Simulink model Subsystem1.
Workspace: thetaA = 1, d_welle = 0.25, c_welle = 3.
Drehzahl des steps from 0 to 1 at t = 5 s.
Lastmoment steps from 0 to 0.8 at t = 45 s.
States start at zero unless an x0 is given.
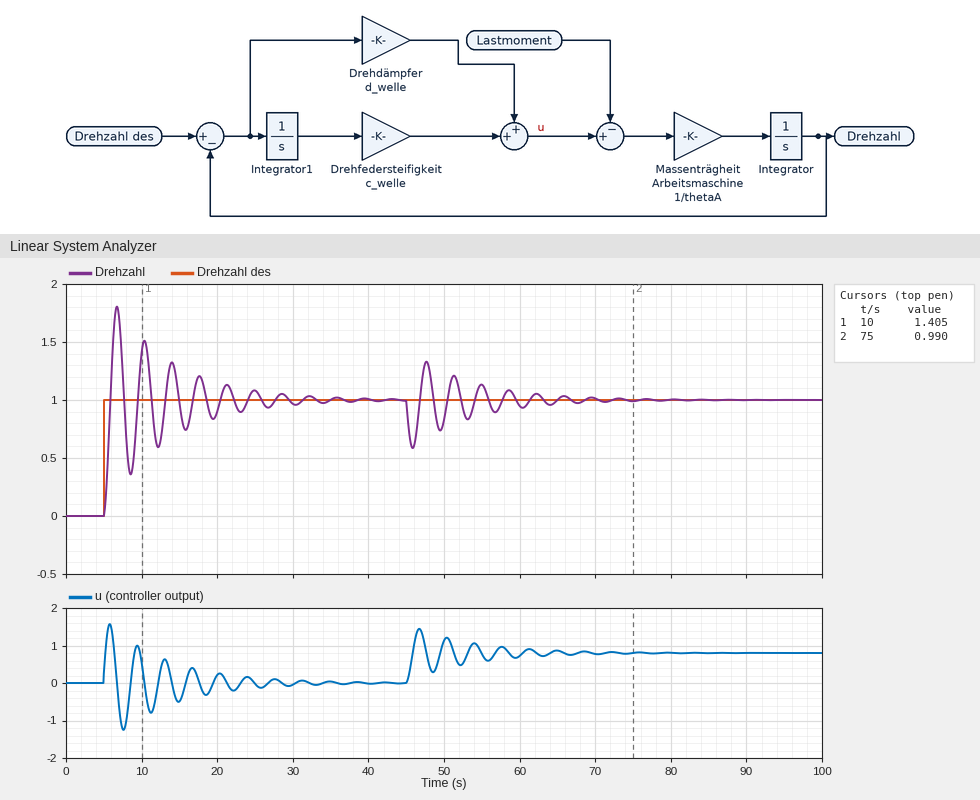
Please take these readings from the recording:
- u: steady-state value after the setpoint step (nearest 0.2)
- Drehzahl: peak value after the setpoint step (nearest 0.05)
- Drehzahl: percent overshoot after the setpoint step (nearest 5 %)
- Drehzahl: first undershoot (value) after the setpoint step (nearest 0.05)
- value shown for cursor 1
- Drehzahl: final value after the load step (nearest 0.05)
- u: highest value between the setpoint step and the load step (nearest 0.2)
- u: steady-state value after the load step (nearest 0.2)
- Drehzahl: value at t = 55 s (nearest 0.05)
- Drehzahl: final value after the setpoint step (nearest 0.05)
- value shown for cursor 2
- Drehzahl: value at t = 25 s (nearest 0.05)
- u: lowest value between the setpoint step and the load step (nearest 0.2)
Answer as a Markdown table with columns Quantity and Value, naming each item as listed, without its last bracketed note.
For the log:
| Quantity | Value |
|---|---|
| u: steady-state value after the setpoint step | 0.0 |
| Drehzahl: peak value after the setpoint step | 1.80 |
| Drehzahl: percent overshoot after the setpoint step | 80 % |
| Drehzahl: first undershoot (value) after the setpoint step | 0.35 |
| value shown for cursor 1 | 1.405 |
| Drehzahl: final value after the load step | 1.00 |
| u: highest value between the setpoint step and the load step | 1.6 |
| u: steady-state value after the load step | 0.8 |
| Drehzahl: value at t = 55 s | 1.15 |
| Drehzahl: final value after the setpoint step | 1.00 |
| value shown for cursor 2 | 0.990 |
| Drehzahl: value at t = 25 s | 1.10 |
| u: lowest value between the setpoint step and the load step | -1.2 |
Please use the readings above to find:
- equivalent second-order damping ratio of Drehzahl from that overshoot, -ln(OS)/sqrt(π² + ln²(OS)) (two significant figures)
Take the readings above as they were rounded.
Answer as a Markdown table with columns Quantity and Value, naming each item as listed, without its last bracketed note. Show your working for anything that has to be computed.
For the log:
| Quantity | Value |
|---|---|
| equivalent second-order damping ratio of Drehzahl from that overshoot, -ln(OS)/sqrt(π² + ln²(OS)) | ln(0.8) = -0.223; 0.223 / sqrt(9.870 + 0.050) = 0.071 |
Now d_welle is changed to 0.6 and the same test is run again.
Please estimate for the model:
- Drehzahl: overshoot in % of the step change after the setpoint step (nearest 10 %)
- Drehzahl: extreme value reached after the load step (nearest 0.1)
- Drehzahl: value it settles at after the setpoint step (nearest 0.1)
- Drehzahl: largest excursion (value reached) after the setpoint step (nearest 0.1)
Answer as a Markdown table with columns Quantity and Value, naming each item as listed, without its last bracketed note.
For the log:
| Quantity | Value |
|---|---|
| Drehzahl: overshoot in % of the step change after the setpoint step | 60 % |
| Drehzahl: extreme value reached after the load step | 0.6 |
| Drehzahl: value it settles at after the setpoint step | 1.0 |
| Drehzahl: largest excursion (value reached) after the setpoint step | 1.6 |
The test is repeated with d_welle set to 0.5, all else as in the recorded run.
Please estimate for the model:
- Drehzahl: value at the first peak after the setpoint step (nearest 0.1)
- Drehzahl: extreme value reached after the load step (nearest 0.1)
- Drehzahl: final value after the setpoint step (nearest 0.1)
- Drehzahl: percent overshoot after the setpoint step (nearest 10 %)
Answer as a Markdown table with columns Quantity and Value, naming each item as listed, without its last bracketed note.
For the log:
| Quantity | Value |
|---|---|
| Drehzahl: value at the first peak after the setpoint step | 1.7 |
| Drehzahl: extreme value reached after the load step | 0.6 |
| Drehzahl: final value after the setpoint step | 1.0 |
| Drehzahl: percent overshoot after the setpoint step | 70 % |
